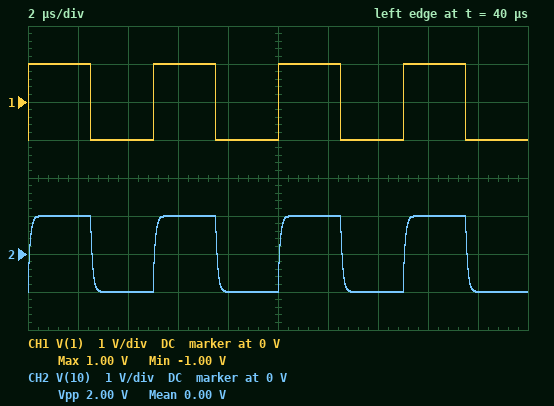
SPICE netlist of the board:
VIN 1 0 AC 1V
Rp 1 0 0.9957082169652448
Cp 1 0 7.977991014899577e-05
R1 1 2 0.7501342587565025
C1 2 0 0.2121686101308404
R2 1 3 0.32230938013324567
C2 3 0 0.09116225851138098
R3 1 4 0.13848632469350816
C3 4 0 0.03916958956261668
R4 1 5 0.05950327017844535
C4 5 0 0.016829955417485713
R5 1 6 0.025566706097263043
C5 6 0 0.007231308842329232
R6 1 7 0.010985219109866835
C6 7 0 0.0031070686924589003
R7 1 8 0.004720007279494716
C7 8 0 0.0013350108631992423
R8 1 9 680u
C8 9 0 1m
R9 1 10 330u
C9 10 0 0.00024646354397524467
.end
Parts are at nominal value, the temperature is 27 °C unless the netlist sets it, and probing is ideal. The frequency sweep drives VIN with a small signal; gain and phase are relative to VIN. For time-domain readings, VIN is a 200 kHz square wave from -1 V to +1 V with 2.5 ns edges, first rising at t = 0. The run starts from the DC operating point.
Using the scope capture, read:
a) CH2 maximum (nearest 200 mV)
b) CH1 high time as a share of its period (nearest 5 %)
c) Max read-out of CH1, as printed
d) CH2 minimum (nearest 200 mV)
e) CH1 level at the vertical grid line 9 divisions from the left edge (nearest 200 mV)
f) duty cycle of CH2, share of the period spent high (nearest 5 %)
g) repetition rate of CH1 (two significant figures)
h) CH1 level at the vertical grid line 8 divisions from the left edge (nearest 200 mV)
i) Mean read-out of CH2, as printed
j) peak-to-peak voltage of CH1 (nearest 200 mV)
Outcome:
1.0 V
50 %
1.00 V
-1.0 V
-1.0 V
50 %
200 kHz
1.0 V
0.00 V
2.0 V
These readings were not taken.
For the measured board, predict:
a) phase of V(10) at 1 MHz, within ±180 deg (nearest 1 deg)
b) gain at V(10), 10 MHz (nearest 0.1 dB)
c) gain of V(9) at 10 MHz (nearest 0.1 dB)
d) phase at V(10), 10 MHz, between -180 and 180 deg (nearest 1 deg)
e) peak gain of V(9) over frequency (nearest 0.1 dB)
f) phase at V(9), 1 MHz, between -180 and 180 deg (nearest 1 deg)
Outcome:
-27 deg
-14.3 dB
-32.6 dB
-79 deg
0 dB
-77 deg
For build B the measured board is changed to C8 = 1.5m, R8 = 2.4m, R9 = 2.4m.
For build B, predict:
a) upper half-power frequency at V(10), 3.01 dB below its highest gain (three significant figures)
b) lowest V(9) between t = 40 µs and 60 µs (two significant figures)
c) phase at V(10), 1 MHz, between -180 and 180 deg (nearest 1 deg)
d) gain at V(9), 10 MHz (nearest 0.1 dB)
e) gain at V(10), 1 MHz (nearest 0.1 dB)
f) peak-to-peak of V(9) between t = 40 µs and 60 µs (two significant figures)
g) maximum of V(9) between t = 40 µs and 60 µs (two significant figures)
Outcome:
269 kHz
-330 mV
-75 deg
-47.1 dB
-11.7 dB
670 mV
330 mV
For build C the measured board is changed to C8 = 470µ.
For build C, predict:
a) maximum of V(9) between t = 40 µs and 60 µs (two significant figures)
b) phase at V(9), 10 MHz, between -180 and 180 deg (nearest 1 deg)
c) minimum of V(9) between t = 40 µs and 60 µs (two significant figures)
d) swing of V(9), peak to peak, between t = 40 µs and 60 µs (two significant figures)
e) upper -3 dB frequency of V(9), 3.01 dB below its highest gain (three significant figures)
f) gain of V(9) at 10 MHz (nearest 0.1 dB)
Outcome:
1.0 V
-87 deg
-1.0 V
2.0 V
498 kHz
-26.1 dB
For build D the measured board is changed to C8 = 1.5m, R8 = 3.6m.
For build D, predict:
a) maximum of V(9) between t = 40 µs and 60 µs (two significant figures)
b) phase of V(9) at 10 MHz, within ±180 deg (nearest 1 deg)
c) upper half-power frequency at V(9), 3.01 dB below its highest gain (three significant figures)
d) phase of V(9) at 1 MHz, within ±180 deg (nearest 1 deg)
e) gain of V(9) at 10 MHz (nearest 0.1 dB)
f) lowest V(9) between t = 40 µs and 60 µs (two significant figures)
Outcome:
230 mV
-90 deg
29.5 kHz
-88 deg
-50.6 dB
-230 mV
